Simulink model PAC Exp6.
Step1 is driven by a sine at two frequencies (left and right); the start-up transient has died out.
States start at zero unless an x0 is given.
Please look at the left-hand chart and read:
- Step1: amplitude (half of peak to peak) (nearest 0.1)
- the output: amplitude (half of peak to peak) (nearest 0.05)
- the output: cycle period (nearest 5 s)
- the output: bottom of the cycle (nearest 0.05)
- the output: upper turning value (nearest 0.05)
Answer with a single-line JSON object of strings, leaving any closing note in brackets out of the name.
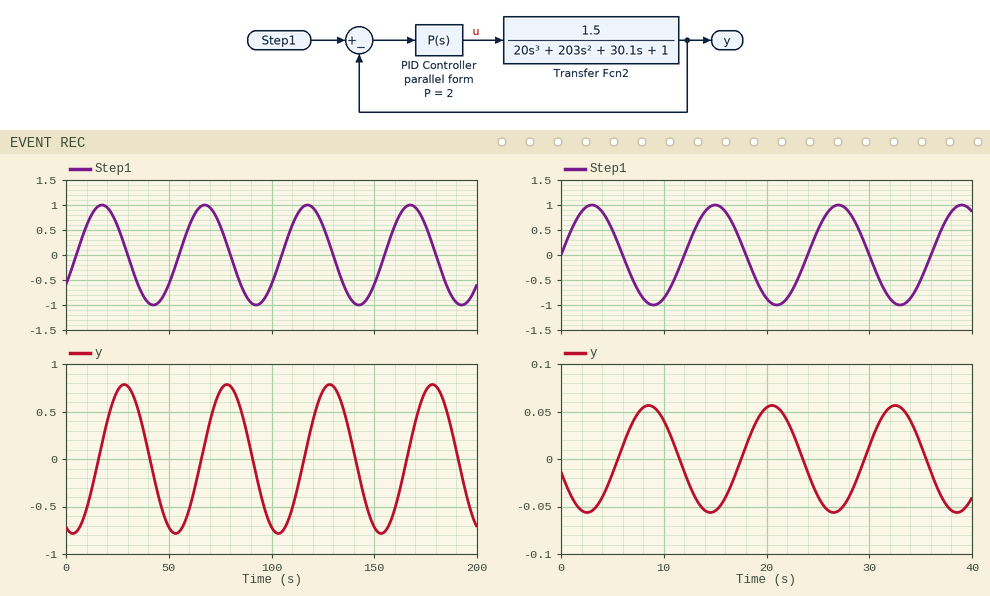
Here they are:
{"Step1: amplitude (half of peak to peak)": "1.0", "the output: amplitude (half of peak to peak)": "0.80", "the output: cycle period": "50 s", "the output: bottom of the cycle": "-0.80", "the output: upper turning value": "0.80"}
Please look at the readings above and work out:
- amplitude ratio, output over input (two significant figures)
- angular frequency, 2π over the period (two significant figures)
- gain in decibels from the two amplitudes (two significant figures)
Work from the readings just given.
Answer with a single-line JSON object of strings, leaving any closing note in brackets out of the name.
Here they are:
{"amplitude ratio, output over input": "0.80", "angular frequency, 2π over the period": "0.13 rad/s", "gain in decibels from the two amplitudes": "-1.9 dB"}
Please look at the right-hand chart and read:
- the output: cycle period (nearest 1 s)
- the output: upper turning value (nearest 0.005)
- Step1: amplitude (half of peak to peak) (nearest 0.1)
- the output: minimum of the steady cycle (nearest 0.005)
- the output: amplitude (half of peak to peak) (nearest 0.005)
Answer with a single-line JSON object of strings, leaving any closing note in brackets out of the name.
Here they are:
{"the output: cycle period": "12 s", "the output: upper turning value": "0.055", "Step1: amplitude (half of peak to peak)": "1.0", "the output: minimum of the steady cycle": "-0.055", "the output: amplitude (half of peak to peak)": "0.055"}
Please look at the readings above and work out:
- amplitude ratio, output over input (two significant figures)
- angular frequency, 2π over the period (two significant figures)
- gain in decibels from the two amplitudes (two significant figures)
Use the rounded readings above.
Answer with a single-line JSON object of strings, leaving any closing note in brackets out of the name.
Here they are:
{"amplitude ratio, output over input": "0.055", "angular frequency, 2π over the period": "0.52 rad/s", "gain in decibels from the two amplitudes": "-25 dB"}
